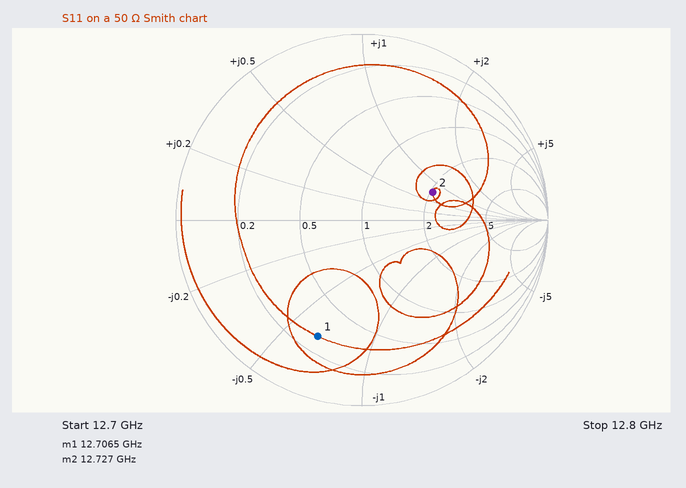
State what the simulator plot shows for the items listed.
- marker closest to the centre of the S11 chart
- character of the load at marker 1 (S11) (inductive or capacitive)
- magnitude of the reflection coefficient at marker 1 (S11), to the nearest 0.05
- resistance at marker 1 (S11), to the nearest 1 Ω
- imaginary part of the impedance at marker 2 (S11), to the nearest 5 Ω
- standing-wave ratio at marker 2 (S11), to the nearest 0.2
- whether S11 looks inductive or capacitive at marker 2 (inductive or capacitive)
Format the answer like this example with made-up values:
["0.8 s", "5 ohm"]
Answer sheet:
["marker 2", "capacitive", "0.65", "14 Ω", "+35 Ω", "2.4", "inductive"]
